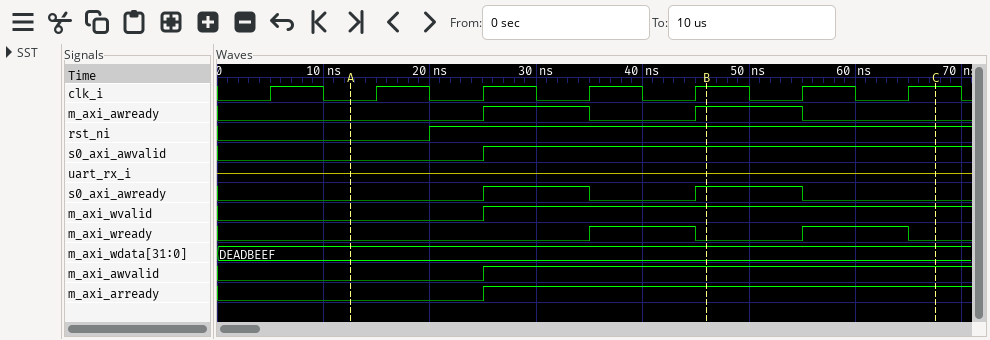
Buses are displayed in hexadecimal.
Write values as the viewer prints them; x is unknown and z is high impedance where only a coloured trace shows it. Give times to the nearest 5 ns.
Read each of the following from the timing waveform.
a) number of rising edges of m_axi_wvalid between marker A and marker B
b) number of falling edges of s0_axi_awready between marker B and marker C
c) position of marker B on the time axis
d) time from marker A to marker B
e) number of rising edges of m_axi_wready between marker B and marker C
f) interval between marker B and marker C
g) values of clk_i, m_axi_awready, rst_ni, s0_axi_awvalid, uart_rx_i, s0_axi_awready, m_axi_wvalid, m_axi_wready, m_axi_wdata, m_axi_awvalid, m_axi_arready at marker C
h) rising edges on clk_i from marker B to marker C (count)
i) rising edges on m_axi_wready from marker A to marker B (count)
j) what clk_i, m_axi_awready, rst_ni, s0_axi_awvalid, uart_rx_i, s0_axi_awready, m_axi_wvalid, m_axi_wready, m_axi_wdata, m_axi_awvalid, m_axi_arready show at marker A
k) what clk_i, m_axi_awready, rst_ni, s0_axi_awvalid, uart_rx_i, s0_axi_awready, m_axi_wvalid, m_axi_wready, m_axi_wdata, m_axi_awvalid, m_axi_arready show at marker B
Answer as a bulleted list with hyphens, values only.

- 1
- 1
- 45 ns
- 35 ns
- 1
- 20 ns
- clk_i=1, m_axi_awready=0, rst_ni=1, s0_axi_awvalid=1, uart_rx_i=z, s0_axi_awready=0, m_axi_wvalid=1, m_axi_wready=0, m_axi_wdata=DEADBEEF, m_axi_awvalid=1, m_axi_arready=1
- 2
- 1
- clk_i=0, m_axi_awready=0, rst_ni=0, s0_axi_awvalid=0, uart_rx_i=z, s0_axi_awready=0, m_axi_wvalid=0, m_axi_wready=0, m_axi_wdata=DEADBEEF, m_axi_awvalid=0, m_axi_arready=0
- clk_i=1, m_axi_awready=1, rst_ni=1, s0_axi_awvalid=1, uart_rx_i=z, s0_axi_awready=1, m_axi_wvalid=1, m_axi_wready=0, m_axi_wdata=DEADBEEF, m_axi_awvalid=1, m_axi_arready=1
